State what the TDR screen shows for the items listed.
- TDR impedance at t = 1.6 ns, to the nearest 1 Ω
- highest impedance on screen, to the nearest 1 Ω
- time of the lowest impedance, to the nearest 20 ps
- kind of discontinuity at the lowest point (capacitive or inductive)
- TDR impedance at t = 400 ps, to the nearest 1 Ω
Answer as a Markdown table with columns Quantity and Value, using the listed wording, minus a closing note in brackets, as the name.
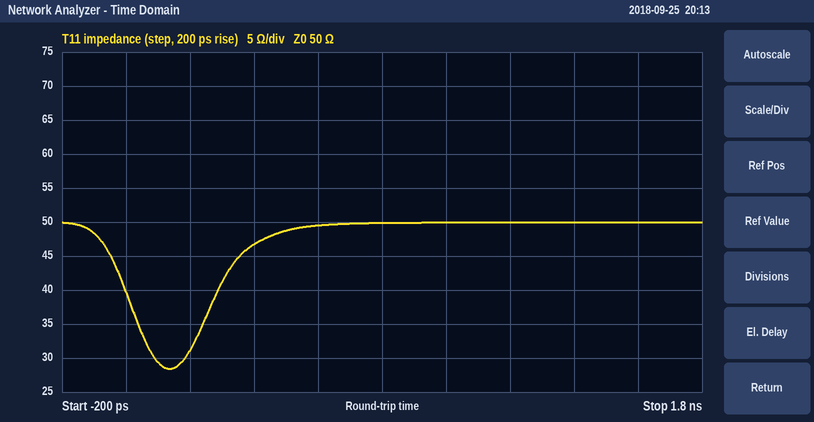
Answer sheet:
| Quantity | Value |
|---|---|
| TDR impedance at t = 1.6 ns, to the nearest 1 Ω | 50 Ω |
| highest impedance on screen, to the nearest 1 Ω | 50 Ω |
| time of the lowest impedance, to the nearest 20 ps | 140 ps |
| kind of discontinuity at the lowest point | capacitive |
| TDR impedance at t = 400 ps, to the nearest 1 Ω | 47 Ω |
